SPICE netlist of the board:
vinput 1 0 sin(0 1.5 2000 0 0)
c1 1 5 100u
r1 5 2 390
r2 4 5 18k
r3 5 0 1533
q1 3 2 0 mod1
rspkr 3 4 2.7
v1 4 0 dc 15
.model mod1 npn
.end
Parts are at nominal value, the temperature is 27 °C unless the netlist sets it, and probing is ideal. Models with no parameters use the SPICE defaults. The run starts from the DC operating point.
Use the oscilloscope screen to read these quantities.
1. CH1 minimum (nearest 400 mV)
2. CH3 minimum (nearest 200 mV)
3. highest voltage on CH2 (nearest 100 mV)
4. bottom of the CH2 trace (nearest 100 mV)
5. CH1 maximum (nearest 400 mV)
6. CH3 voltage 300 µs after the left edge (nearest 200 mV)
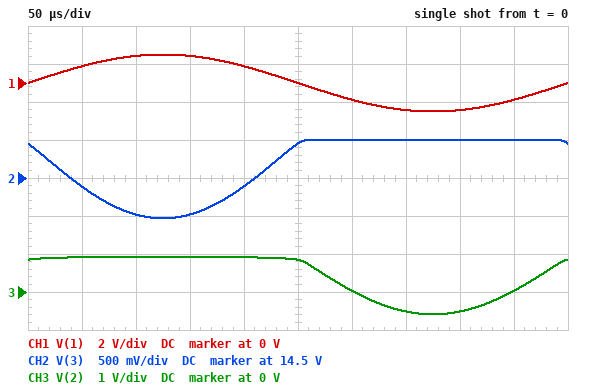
-1.6 V
-600 mV
15.0 V
14.0 V
1.6 V
0 V
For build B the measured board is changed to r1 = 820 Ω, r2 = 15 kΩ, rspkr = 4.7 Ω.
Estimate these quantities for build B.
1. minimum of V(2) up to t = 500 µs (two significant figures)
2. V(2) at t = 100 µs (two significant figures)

-450 mV
910 mV
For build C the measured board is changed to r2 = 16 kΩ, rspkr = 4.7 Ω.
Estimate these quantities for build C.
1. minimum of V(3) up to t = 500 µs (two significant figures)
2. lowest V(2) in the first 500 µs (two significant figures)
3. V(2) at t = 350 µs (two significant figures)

13 V
-550 mV
-480 mV
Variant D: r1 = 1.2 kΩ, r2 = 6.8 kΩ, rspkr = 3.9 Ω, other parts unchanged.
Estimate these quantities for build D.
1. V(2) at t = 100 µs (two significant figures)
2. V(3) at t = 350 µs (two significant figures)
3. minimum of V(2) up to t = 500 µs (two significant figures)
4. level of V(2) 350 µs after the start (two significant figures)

910 mV
15 V
300 mV
370 mV
